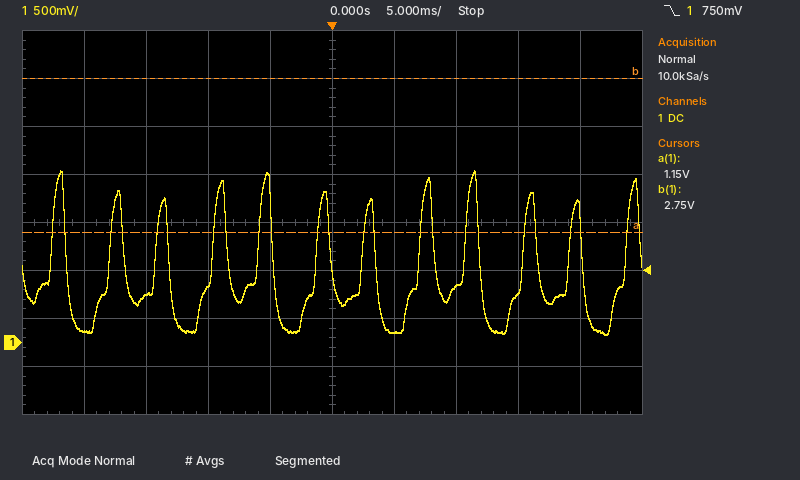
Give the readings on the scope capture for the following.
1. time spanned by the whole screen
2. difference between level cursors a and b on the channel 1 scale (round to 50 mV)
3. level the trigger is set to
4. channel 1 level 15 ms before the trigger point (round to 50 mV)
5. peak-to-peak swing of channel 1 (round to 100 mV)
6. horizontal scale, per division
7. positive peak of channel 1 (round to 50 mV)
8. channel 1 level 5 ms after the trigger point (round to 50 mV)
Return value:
50 ms
1.60 V
750 mV
500 mV
1.70 V
5 ms
1.80 V
100 mV
